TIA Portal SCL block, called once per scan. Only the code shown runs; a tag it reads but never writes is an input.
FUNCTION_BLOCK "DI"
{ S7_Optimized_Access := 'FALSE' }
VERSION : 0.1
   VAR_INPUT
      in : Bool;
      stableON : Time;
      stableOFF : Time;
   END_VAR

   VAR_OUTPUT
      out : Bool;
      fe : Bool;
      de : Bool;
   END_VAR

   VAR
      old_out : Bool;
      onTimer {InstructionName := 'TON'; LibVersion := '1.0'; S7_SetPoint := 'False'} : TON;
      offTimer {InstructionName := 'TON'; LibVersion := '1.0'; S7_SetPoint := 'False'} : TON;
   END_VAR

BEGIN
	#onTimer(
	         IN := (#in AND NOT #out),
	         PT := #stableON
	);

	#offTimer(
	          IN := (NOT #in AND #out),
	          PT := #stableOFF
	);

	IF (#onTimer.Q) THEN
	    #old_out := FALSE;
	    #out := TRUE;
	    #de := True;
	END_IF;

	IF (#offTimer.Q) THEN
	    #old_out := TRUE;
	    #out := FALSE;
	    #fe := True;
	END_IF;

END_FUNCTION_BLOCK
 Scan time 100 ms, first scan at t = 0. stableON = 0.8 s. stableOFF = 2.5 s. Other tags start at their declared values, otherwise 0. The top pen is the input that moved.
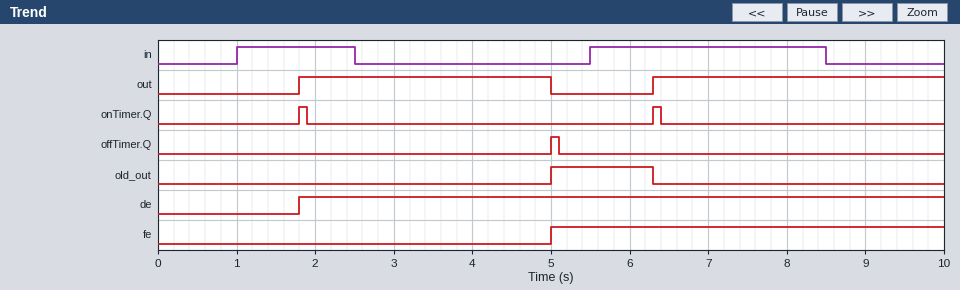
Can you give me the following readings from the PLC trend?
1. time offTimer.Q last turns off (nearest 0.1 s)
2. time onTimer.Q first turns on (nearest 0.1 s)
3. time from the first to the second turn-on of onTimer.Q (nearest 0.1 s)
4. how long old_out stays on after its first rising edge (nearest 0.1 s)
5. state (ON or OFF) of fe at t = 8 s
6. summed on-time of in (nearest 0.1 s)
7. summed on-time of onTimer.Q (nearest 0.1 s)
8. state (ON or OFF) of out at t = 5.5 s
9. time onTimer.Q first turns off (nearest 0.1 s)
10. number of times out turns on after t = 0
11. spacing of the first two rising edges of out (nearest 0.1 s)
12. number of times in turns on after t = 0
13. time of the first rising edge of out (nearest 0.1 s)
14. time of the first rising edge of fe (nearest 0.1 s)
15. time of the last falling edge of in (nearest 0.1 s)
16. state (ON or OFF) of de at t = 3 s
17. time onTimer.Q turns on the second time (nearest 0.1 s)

5.1 s
1.8 s
4.5 s
1.3 s
ON
4.5 s
0.2 s
OFF
1.9 s
2
4.5 s
2
1.8 s
5.0 s
8.5 s
ON
6.3 s
